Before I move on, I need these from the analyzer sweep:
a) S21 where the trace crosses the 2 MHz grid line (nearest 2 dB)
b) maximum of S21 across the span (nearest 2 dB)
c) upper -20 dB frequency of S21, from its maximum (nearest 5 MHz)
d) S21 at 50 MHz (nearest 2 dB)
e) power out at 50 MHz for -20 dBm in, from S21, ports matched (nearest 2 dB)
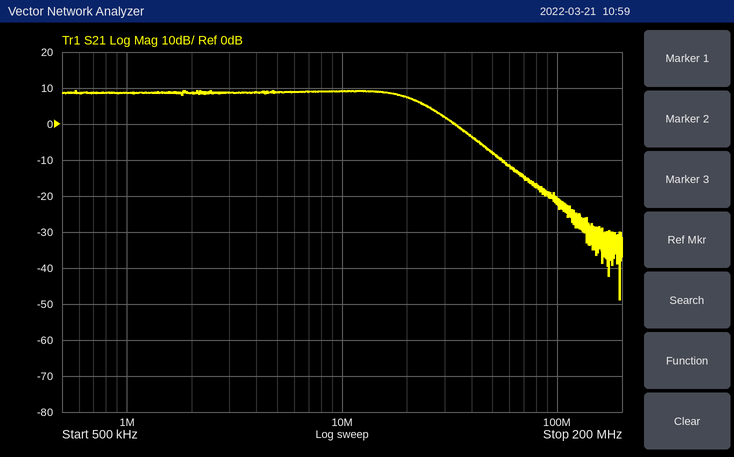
8 dB
10 dB
55 MHz
-8 dB
-28 dBm
